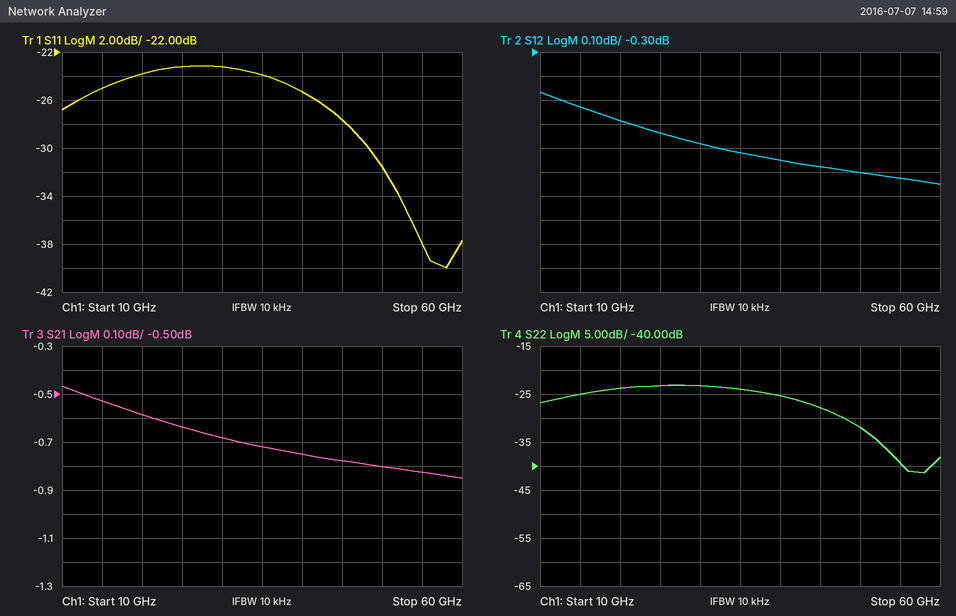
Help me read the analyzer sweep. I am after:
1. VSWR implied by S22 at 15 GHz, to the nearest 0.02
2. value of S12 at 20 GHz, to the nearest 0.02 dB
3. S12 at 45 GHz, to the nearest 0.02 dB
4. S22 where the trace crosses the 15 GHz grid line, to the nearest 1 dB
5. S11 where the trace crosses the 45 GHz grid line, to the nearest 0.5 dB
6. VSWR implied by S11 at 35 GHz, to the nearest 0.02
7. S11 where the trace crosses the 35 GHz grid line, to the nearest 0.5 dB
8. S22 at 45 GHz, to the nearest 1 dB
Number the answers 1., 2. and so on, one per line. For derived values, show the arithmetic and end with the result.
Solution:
1. |Γ| = 10^(-25/20) = 0.0562; VSWR = (1 + 0.0562)/(1 − 0.0562) ≈ 1.12
2. -0.58 dB
3. -0.78 dB
4. -25 dB
5. -27.5 dB
6. |Γ| = 10^(-24/20) = 0.0631; VSWR = (1 + 0.0631)/(1 − 0.0631) ≈ 1.13, so 1.14 to the nearest 0.02
7. -24.0 dB
8. -28 dB
